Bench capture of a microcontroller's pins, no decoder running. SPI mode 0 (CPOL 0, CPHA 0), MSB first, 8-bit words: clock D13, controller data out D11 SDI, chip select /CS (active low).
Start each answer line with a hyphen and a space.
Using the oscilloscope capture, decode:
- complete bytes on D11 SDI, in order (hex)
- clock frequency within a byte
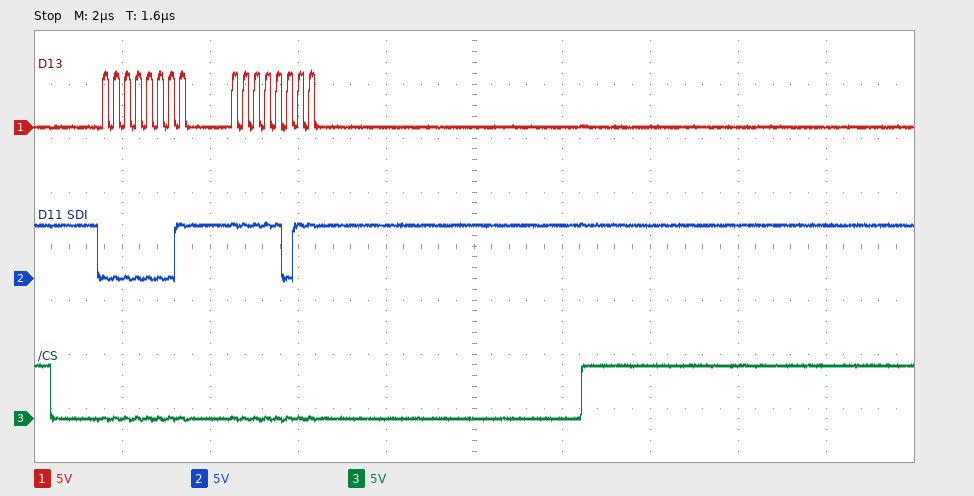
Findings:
- 01 FB
- 4 MHz
